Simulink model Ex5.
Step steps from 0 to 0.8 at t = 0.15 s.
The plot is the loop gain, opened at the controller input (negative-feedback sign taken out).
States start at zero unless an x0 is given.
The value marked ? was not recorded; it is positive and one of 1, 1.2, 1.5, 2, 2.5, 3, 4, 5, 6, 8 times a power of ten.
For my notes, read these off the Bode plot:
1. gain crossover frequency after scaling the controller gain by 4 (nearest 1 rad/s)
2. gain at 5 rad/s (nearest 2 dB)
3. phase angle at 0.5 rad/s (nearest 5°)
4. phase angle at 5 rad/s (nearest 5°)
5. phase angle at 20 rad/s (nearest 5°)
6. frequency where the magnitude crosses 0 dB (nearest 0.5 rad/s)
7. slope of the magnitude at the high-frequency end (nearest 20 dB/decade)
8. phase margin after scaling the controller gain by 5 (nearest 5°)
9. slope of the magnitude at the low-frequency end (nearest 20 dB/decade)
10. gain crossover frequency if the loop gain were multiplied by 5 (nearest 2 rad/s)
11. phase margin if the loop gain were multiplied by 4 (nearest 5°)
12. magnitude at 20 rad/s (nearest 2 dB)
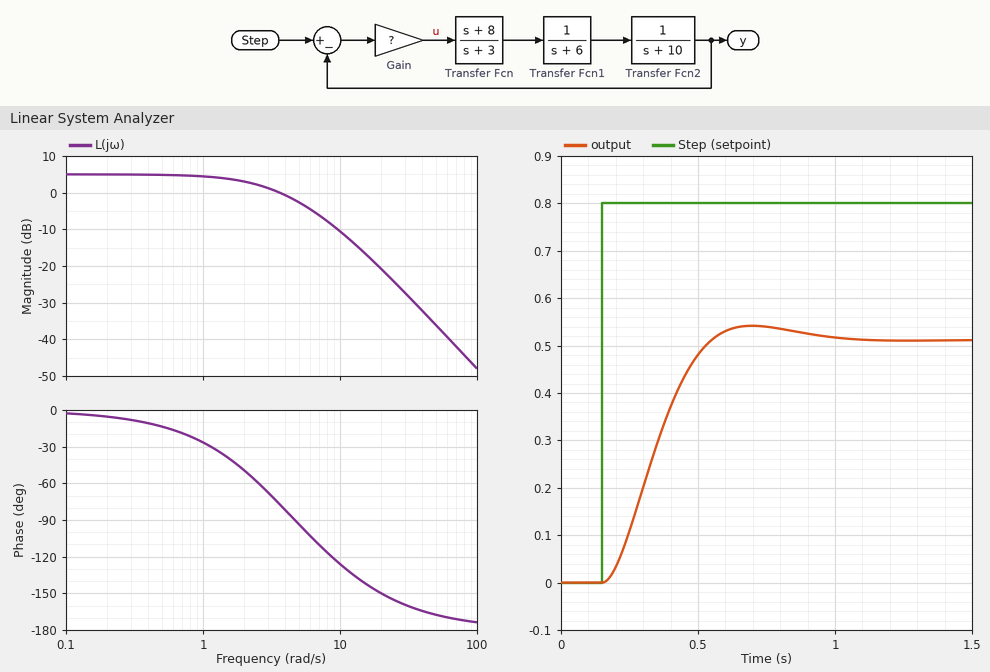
11 rad/s
-2 dB
-15°
-95°
-150°
3.5 rad/s
-40 dB/decade
45°
0 dB/decade
12 rad/s
50°
-20 dB
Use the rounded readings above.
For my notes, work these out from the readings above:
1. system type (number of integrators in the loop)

0
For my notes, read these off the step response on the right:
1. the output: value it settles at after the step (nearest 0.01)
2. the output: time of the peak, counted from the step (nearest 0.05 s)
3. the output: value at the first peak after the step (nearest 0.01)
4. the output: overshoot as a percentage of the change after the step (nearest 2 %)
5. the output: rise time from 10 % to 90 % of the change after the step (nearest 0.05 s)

0.51
0.55 s
0.54
6 %
0.25 s
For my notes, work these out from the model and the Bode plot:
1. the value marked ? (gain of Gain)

40
